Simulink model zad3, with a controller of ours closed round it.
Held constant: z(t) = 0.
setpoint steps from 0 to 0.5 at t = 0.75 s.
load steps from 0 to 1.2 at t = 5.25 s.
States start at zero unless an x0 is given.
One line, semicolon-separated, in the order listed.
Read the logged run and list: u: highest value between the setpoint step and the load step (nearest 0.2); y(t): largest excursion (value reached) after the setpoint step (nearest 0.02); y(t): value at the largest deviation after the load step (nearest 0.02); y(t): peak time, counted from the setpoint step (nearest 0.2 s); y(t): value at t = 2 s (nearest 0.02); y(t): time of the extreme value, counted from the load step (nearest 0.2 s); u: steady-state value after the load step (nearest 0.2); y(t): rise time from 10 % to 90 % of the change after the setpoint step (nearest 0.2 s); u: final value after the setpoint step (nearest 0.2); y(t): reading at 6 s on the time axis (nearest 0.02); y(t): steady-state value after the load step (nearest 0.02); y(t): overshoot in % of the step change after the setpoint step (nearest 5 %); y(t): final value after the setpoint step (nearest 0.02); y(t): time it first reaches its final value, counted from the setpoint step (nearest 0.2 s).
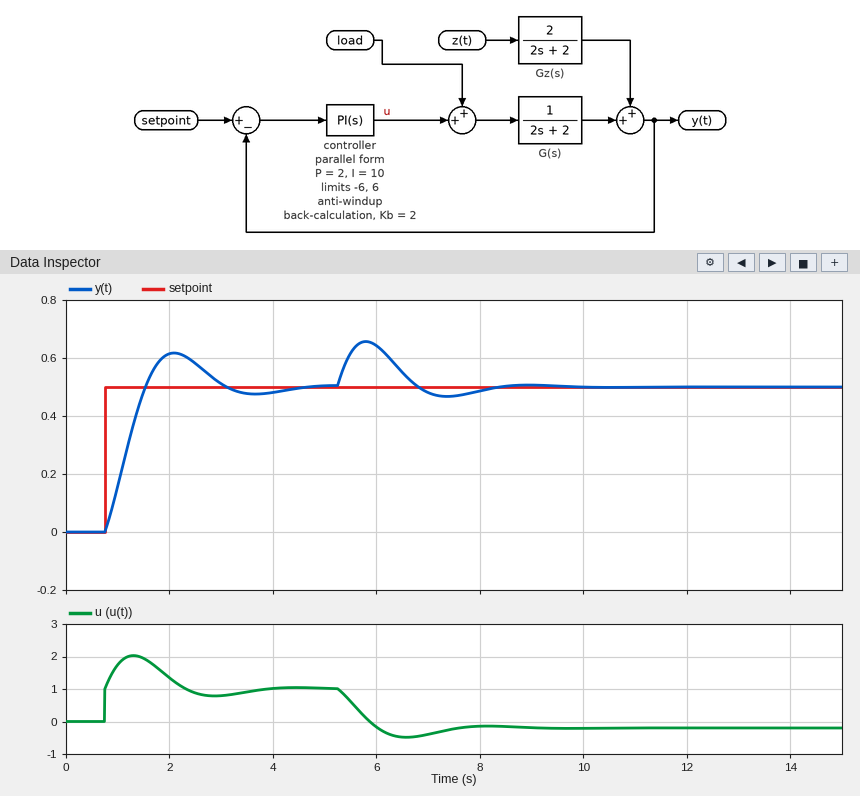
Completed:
2.0; 0.62; 0.66; 1.4 s; 0.62; 0.6 s; -0.2; 0.6 s; 1.0; 0.64; 0.50; 25 %; 0.50; 0.8 s
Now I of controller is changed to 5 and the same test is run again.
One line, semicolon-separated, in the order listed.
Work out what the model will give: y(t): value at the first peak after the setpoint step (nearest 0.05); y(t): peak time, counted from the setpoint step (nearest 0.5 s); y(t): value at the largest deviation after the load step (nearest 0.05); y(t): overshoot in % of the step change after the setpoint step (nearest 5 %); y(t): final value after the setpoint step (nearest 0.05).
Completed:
0.55; 2.0 s; 0.70; 10 %; 0.50
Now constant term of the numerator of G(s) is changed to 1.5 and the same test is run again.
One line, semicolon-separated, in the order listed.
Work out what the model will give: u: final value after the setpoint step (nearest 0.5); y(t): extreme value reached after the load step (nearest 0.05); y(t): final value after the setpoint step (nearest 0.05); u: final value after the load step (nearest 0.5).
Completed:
0.5; 0.70; 0.50; -0.5
